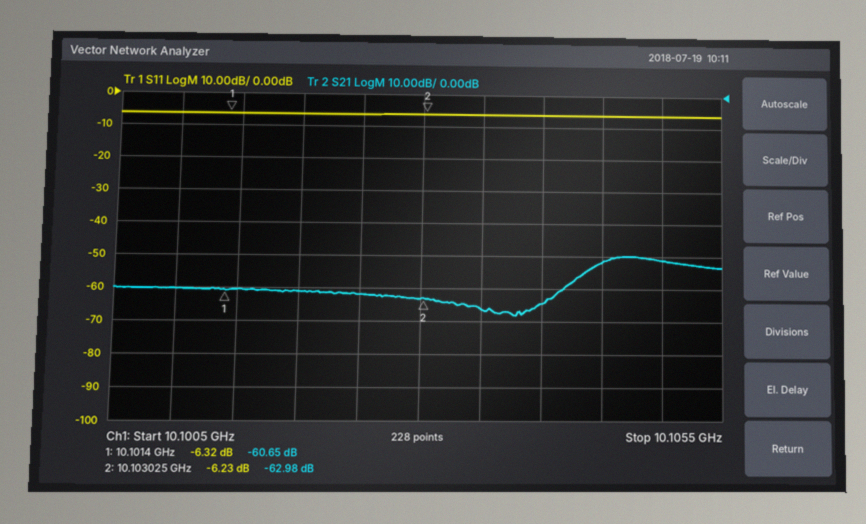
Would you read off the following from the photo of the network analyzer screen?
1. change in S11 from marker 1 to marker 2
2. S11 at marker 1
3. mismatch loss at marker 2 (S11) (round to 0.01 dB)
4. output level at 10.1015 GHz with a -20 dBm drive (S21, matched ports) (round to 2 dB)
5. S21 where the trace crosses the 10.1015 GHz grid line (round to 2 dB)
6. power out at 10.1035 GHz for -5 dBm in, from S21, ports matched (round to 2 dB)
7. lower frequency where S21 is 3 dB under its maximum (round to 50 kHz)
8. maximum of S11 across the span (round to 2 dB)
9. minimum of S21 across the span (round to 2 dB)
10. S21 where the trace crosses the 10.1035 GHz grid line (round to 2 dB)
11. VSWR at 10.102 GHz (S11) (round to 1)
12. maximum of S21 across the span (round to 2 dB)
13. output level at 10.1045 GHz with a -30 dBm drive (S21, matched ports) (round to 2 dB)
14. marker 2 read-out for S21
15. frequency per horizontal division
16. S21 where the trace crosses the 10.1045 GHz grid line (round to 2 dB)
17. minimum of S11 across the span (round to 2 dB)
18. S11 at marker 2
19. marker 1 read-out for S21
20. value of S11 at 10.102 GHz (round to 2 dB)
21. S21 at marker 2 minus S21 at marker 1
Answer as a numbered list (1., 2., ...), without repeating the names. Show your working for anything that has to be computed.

1. -6.23 − (-6.32) = 0.09 dB
2. -6.32 dB
3. −10 log10(1 − 10^(-6.23/10)) ≈ 1.18 dB
4. -20 dBm + (-60 dB) = -80 dBm
5. -60 dB
6. -5 dBm + (-66 dB) = -72 dBm
7. 10.10445 GHz
8. -6 dB
9. -68 dB
10. -66 dB
11. |Γ| = 10^(-6/20) = 0.5012; VSWR = (1 + 0.5012)/(1 − 0.5012) ≈ 3
12. -50 dB
13. -30 dBm + (-52 dB) = -82 dBm
14. -62.98 dB
15. 500 kHz
16. -52 dB
17. -6 dB
18. -6.23 dB
19. -60.65 dB
20. -6 dB
21. -62.98 − (-60.65) = -2.33 dB
